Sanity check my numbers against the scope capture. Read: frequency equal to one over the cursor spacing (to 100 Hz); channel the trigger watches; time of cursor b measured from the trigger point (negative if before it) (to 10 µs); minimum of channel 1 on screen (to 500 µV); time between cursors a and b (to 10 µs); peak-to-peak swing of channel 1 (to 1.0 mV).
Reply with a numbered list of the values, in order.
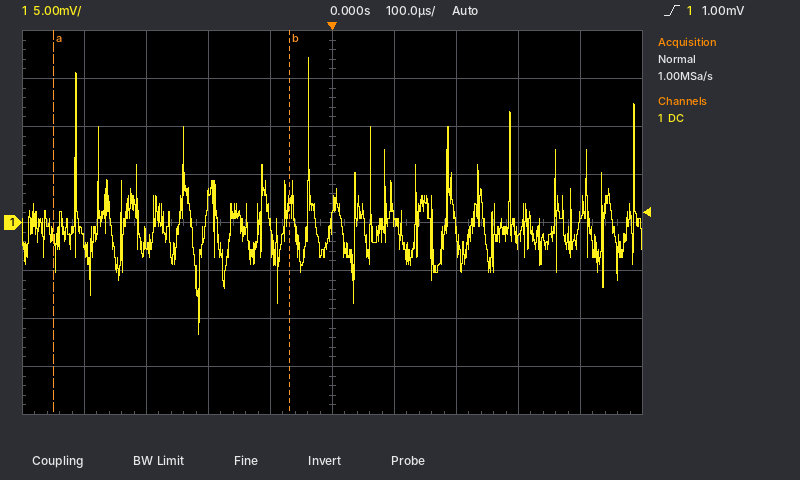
1. 2.6 kHz
2. channel 1
3. -70 µs
4. -11.5 mV
5. 380 µs
6. 29.0 mV
